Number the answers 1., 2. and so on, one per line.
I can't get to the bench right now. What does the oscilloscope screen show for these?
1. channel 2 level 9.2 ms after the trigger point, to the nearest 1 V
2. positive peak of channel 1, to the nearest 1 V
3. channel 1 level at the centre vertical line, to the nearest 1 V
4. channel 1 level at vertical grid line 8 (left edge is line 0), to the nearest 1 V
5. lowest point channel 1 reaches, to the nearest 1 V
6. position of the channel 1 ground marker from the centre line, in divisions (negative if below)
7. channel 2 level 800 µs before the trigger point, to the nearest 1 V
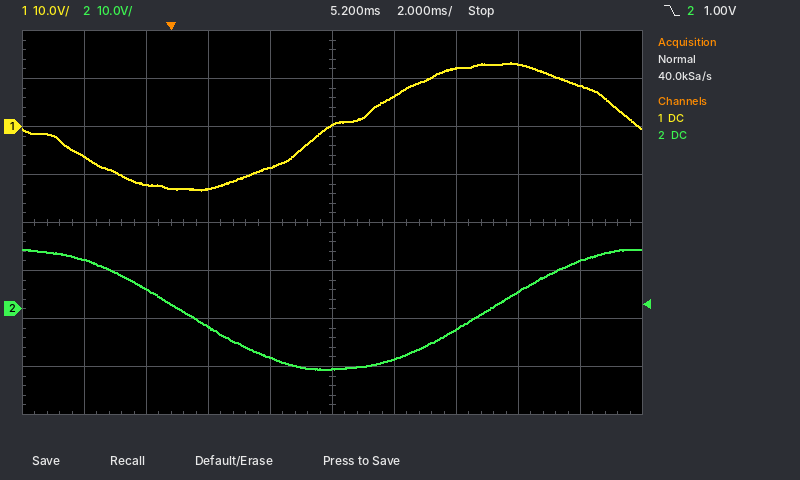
1. -4 V
2. 13 V
3. 0 V
4. 13 V
5. -13 V
6. +2.0 div
7. 4 V
